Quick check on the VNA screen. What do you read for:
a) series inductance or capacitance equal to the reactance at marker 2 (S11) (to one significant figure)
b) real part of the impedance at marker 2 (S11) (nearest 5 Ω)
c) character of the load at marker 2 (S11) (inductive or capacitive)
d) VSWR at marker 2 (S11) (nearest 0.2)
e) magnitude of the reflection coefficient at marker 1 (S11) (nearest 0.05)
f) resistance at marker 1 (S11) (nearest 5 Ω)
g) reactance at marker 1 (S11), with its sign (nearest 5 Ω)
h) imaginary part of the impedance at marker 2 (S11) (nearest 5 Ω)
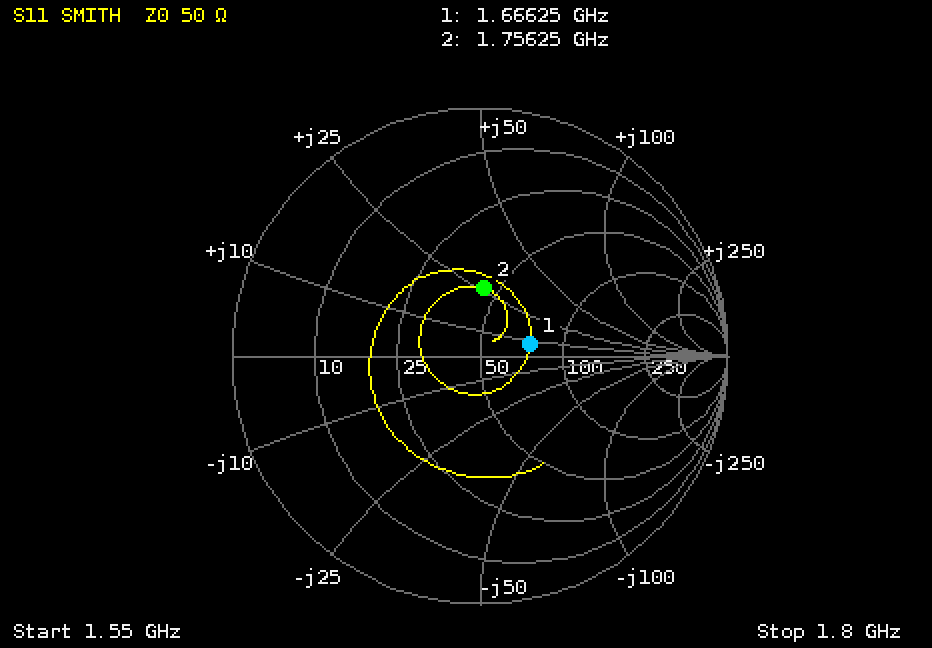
2 nH
45 Ω
inductive
1.8
0.20
75 Ω
+10 Ω
+25 Ω
